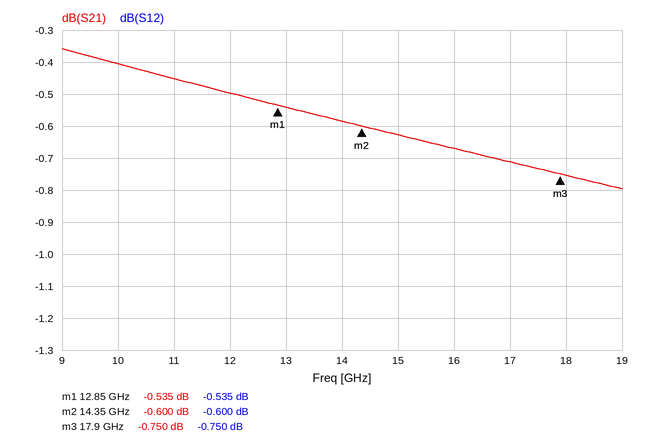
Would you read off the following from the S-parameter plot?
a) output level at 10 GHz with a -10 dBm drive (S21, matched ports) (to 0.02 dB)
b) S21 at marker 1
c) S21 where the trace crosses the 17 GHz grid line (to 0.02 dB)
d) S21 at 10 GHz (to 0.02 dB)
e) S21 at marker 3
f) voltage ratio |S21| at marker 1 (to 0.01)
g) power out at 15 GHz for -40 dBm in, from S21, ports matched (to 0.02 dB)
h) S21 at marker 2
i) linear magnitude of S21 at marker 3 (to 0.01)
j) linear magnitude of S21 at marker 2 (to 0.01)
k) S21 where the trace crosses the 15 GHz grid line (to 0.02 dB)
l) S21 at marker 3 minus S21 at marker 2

-10.40 dBm
-0.535 dB
-0.72 dB
-0.40 dB
-0.750 dB
0.94
-40.62 dBm
-0.600 dB
0.92
0.93
-0.62 dB
-0.150 dB
